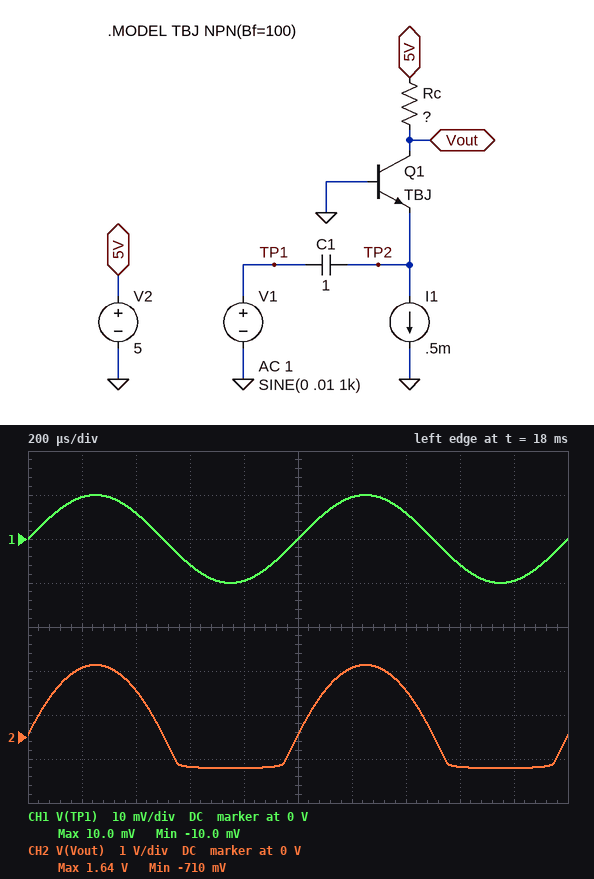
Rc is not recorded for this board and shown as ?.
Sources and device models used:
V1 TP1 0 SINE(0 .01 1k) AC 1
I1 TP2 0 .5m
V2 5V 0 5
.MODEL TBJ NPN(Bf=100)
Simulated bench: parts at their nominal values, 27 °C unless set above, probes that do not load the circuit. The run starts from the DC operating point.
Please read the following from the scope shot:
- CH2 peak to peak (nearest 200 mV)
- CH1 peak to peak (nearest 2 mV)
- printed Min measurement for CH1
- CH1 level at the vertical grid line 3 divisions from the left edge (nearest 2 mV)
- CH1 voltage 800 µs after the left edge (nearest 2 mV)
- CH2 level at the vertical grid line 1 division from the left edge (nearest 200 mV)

2.4 V
20 mV
-10.0 mV
-6 mV
-10 mV
1.6 V
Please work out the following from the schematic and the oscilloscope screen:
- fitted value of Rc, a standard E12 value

10 kΩ
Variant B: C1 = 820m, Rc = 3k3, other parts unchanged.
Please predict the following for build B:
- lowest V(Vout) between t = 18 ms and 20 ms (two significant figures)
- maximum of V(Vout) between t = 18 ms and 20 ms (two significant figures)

2.6 V
3.9 V
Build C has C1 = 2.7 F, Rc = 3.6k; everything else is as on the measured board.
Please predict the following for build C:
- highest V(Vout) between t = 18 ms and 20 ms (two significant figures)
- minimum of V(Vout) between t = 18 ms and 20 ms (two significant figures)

3.8 V
2.4 V
